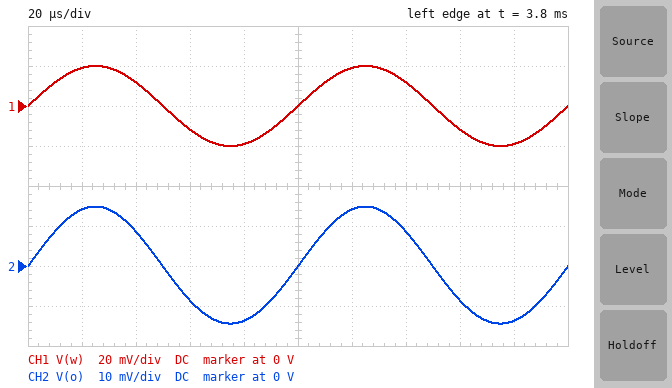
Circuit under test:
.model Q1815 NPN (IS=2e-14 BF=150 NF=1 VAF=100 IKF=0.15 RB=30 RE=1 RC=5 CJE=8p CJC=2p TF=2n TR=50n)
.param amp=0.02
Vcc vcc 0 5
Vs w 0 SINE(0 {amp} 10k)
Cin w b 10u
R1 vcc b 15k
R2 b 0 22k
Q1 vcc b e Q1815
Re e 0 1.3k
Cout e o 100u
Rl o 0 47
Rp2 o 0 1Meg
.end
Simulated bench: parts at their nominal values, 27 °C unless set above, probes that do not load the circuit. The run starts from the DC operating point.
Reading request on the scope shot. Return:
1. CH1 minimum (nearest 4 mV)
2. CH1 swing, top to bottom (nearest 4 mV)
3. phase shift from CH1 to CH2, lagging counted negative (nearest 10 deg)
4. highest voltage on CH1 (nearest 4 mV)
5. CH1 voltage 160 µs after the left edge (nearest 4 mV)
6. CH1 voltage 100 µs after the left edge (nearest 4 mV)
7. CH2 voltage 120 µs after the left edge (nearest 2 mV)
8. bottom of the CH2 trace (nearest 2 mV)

-20 mV
40 mV
0 deg
20 mV
-12 mV
0 V
14 mV
-14 mV
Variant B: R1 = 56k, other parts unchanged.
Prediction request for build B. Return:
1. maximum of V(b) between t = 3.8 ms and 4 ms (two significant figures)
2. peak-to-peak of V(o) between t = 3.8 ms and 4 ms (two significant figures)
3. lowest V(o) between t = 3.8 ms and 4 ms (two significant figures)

1.4 V
19 mV
-8.9 mV
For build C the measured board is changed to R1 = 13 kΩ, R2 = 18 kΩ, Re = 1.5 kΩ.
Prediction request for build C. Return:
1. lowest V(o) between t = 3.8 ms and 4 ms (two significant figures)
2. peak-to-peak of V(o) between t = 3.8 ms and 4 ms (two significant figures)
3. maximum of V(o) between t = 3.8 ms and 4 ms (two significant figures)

-14 mV
28 mV
14 mV
